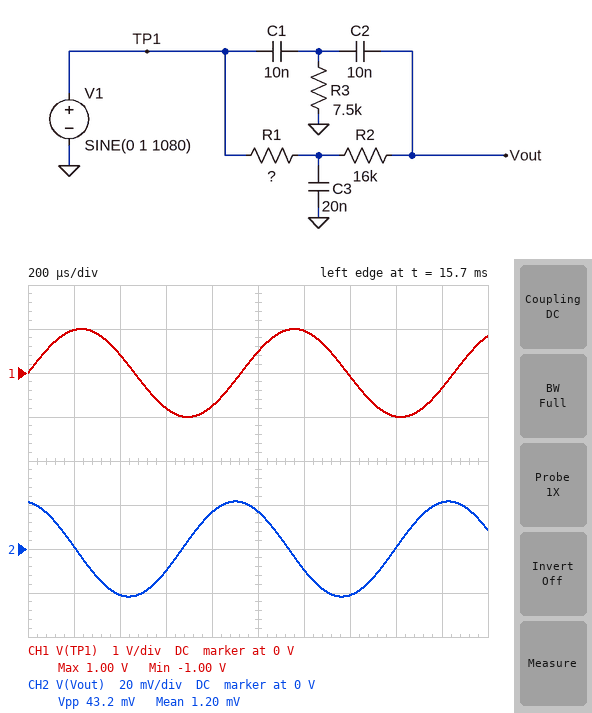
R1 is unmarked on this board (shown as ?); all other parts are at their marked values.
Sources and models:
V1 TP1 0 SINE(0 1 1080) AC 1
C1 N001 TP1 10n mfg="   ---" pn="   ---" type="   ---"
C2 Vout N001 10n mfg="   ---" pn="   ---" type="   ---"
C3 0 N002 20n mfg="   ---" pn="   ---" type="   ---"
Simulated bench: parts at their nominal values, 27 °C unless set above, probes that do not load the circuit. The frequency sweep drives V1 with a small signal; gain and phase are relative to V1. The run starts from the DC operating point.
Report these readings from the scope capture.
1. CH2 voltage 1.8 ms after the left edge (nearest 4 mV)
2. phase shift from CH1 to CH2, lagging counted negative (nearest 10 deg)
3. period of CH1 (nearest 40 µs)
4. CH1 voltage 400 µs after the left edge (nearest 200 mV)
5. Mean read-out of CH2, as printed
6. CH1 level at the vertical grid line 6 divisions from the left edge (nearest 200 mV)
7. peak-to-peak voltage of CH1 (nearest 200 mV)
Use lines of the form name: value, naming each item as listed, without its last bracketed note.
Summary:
CH2 voltage 1.8 ms after the left edge: 20 mV
phase shift from CH1 to CH2, lagging counted negative: 100 deg
period of CH1: 920 µs
CH1 voltage 400 µs after the left edge: 400 mV
Mean read-out of CH2, as printed: 1.20 mV
CH1 level at the vertical grid line 6 divisions from the left edge: 1.0 V
peak-to-peak voltage of CH1: 2.0 V
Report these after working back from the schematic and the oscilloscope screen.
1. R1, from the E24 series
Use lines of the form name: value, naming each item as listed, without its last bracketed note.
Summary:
R1, from the E24 series: 15 kΩ
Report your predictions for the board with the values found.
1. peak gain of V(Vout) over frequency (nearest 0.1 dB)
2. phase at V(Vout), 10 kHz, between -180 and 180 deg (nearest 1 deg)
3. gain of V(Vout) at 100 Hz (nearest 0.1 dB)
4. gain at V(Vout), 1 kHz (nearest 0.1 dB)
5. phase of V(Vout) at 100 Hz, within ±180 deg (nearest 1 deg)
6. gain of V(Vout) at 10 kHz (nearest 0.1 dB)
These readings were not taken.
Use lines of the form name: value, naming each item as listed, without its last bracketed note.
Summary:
peak gain of V(Vout) over frequency: 0 dB
phase at V(Vout), 10 kHz, between -180 and 180 deg: 23 deg
gain of V(Vout) at 100 Hz: -0.6 dB
gain at V(Vout), 1 kHz: -34.8 dB
phase of V(Vout) at 100 Hz, within ±180 deg: -21 deg
gain of V(Vout) at 10 kHz: -0.7 dB
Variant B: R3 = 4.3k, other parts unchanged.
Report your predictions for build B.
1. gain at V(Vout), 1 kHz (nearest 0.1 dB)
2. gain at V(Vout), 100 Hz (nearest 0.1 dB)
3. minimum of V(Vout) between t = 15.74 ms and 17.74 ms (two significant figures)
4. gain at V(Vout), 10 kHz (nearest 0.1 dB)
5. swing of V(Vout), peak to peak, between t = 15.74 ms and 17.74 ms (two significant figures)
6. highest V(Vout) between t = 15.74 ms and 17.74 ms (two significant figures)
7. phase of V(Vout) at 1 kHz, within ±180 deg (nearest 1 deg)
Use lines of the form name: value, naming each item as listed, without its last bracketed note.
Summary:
gain at V(Vout), 1 kHz: -19.7 dB
gain at V(Vout), 100 Hz: -0.5 dB
minimum of V(Vout) between t = 15.74 ms and 17.74 ms: -77 mV
gain at V(Vout), 10 kHz: -1.1 dB
swing of V(Vout), peak to peak, between t = 15.74 ms and 17.74 ms: 150 mV
highest V(Vout) between t = 15.74 ms and 17.74 ms: 77 mV
phase of V(Vout) at 1 kHz, within ±180 deg: -119 deg
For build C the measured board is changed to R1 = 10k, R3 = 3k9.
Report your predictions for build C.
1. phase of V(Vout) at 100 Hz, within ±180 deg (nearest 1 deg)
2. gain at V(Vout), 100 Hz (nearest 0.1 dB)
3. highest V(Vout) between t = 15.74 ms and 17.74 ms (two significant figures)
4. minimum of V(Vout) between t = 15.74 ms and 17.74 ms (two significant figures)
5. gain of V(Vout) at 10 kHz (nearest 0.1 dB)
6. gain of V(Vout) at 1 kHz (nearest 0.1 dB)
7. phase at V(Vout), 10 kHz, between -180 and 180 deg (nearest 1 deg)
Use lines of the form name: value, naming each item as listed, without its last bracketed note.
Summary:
phase of V(Vout) at 100 Hz, within ±180 deg: -16 deg
gain at V(Vout), 100 Hz: -0.3 dB
highest V(Vout) between t = 15.74 ms and 17.74 ms: 150 mV
minimum of V(Vout) between t = 15.74 ms and 17.74 ms: -150 mV
gain of V(Vout) at 10 kHz: -1.3 dB
gain of V(Vout) at 1 kHz: -14.5 dB
phase at V(Vout), 10 kHz, between -180 and 180 deg: 32 deg
